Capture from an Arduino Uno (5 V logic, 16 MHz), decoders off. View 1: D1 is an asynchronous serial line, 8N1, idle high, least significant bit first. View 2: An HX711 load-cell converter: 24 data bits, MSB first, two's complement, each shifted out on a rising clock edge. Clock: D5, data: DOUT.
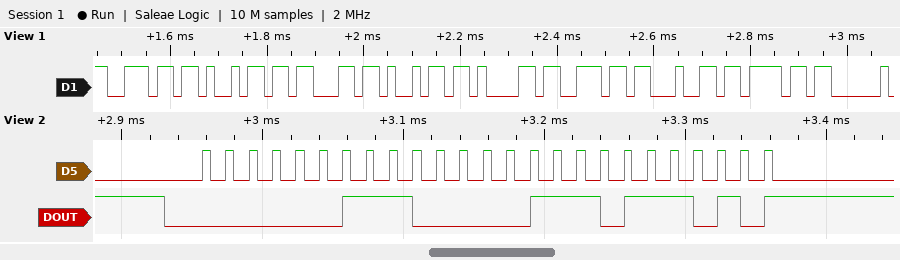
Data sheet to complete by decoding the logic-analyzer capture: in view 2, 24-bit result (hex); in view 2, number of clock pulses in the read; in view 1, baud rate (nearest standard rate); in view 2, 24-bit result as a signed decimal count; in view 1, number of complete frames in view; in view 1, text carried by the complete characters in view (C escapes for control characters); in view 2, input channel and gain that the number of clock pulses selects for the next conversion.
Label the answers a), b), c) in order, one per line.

a) 0x0383BA
b) 25
c) 57600 baud
d) 230330
e) 8
f) "niciando"
g) channel A, gain 128
